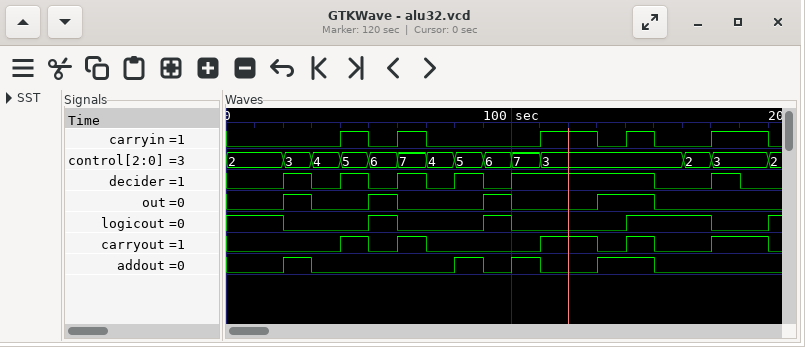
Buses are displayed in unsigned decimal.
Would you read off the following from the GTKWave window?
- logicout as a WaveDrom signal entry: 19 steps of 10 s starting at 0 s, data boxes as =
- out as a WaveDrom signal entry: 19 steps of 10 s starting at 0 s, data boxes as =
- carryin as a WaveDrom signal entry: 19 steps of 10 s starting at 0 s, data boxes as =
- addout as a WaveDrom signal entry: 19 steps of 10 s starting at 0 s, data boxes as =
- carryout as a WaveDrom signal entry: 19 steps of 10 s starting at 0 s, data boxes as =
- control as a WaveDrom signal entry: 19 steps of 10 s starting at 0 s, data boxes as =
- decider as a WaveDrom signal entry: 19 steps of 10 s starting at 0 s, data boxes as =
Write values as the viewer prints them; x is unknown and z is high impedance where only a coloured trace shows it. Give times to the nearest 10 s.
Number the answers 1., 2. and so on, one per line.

1. {name: 'logicout', wave: '1.0..10..10...1..0.'}
2. {name: 'out', wave: '0.10.10..10..1.0...'}
3. {name: 'carryin', wave: '0...1010...1.010.1.'}
4. {name: 'addout', wave: '0.10....1010.1.0...'}
5. {name: 'carryout', wave: '0...1010...1.010.1.'}
6. {name: 'control', wave: '=.==========....==.', data: '2 3 4 5 6 7 4 5 6 7 3 2 3'}
7. {name: 'decider', wave: '0.101010101....0.10'}
